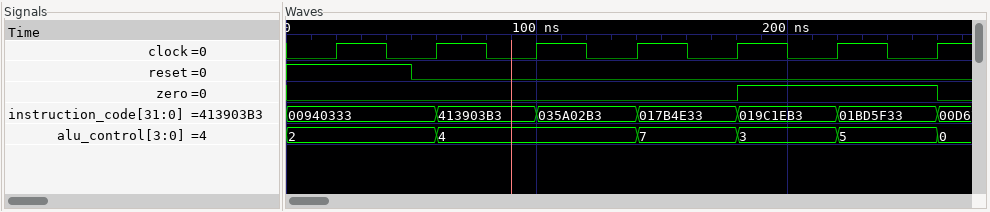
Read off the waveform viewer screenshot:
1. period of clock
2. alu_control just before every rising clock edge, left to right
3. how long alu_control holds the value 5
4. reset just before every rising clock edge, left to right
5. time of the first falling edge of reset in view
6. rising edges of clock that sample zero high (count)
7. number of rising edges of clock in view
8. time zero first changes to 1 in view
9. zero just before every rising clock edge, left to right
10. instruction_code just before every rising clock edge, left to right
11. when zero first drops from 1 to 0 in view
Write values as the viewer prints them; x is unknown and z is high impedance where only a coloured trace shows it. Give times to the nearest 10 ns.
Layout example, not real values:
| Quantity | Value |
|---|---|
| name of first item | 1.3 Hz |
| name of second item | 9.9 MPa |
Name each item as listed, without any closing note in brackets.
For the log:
| Quantity | Value |
|---|---|
| period of clock | 40 ns |
| alu_control just before every rising clock edge, left to right | 2, 2, 4, 4, 7, 3, 5 |
| how long alu_control holds the value 5 | 40 ns |
| reset just before every rising clock edge, left to right | 1 0 0 0 0 0 0 |
| time of the first falling edge of reset in view | 50 ns |
| rising edges of clock that sample zero high | 2 |
| number of rising edges of clock in view | 7 |
| time zero first changes to 1 in view | 180 ns |
| zero just before every rising clock edge, left to right | 0 0 0 0 0 1 1 |
| instruction_code just before every rising clock edge, left to right | 00940333, 00940333, 413903B3, 035A02B3, 017B4E33, 019C1EB3, 01BD5F33 |
| when zero first drops from 1 to 0 in view | 260 ns |
